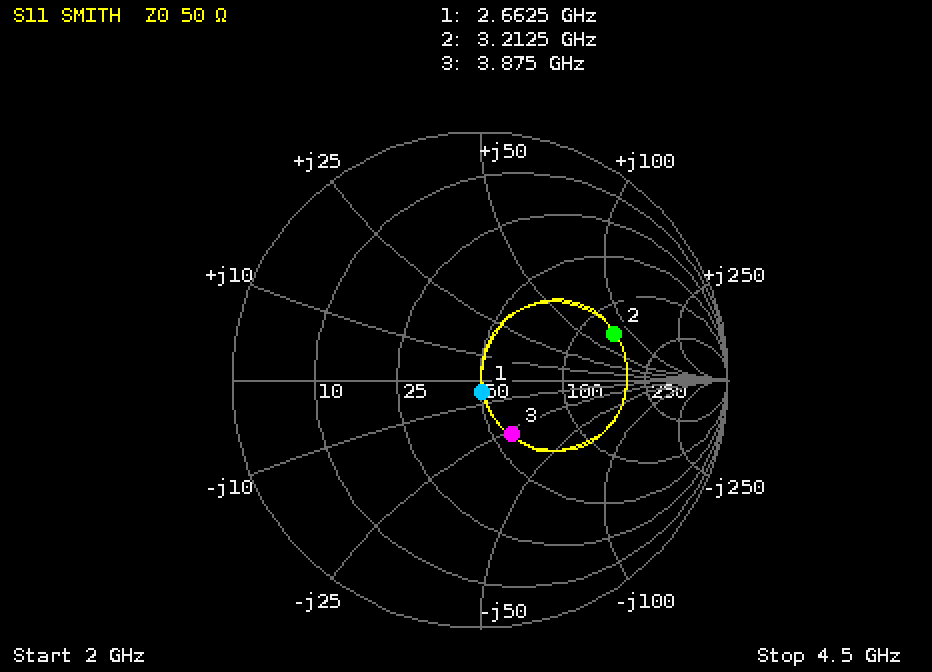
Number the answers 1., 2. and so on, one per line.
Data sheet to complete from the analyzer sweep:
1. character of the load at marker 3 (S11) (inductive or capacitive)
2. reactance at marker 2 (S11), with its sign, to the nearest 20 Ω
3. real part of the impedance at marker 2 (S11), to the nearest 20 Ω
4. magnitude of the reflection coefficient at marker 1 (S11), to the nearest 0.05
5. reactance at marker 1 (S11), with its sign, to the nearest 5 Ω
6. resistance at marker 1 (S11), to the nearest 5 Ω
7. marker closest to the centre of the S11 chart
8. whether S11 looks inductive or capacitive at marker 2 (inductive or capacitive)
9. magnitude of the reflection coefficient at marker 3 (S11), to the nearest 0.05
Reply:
1. capacitive
2. +80 Ω
3. 140 Ω
4. 0.05
5. -5 Ω
6. 50 Ω
7. marker 1
8. inductive
9. 0.25
